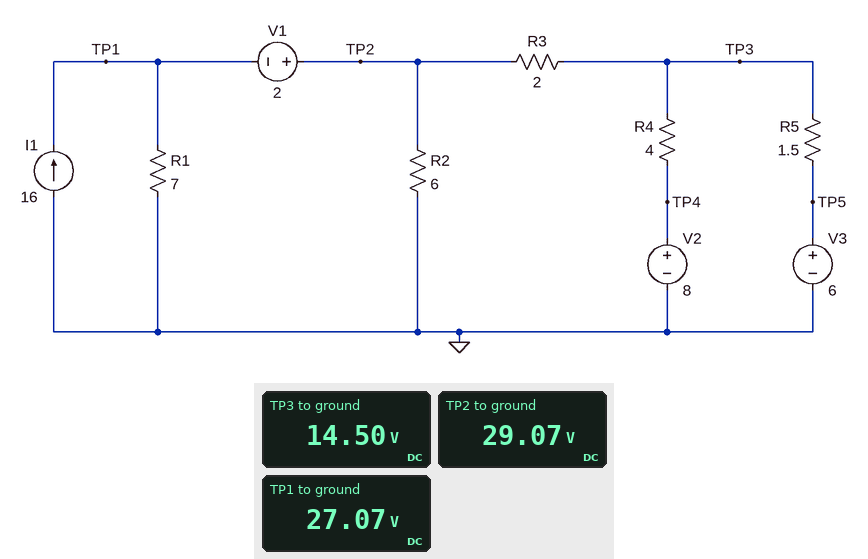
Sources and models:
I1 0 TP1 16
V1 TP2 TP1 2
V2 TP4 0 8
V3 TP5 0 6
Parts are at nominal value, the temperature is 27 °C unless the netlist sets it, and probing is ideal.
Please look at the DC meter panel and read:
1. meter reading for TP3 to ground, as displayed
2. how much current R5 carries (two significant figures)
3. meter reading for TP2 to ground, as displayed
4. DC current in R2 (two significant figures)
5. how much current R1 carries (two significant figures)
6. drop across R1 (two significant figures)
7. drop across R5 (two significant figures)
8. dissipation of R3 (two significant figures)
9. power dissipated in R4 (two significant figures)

14.50 V
5.7 A
29.07 V
4.8 A
3.9 A
27 V
8.5 V
110 W
11 W
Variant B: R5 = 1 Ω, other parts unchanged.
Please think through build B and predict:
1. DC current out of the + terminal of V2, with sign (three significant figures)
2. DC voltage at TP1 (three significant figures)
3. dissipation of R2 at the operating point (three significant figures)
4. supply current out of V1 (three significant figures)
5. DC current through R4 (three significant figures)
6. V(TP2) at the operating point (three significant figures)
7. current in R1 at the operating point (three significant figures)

-1.13 A
25.9 V
129 W
12.3 A
1.13 A
27.9 V
3.69 A
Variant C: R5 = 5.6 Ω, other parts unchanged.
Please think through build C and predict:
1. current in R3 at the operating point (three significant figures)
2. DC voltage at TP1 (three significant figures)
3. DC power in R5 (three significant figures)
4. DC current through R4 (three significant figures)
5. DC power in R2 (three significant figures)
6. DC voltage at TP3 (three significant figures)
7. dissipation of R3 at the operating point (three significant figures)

6.01 A
31.2 V
41.2 W
3.30 A
184 W
21.2 V
72.2 W
